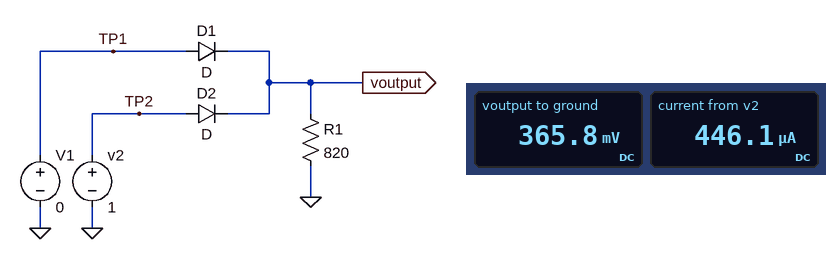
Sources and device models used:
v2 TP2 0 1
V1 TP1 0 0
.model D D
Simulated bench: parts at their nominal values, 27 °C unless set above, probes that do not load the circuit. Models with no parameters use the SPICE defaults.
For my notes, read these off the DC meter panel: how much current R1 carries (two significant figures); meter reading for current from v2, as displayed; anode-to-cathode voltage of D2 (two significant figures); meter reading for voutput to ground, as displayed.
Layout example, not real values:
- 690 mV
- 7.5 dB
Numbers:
- 450 µA
- 446.1 µA
- 630 mV
- 365.8 mV
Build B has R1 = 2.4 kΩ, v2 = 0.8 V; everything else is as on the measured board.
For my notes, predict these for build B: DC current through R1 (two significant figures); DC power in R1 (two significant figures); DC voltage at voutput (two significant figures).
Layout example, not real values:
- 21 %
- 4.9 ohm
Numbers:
- 87 µA
- 18 µW
- 210 mV
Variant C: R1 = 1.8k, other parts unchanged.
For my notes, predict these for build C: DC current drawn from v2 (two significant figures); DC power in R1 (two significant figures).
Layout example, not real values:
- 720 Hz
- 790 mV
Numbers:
- 210 µA
- 82 µW
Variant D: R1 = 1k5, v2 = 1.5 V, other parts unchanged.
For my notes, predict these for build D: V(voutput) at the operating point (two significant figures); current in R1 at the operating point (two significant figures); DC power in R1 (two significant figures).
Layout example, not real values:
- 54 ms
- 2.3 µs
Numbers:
- 860 mV
- 570 µA
- 490 µW
